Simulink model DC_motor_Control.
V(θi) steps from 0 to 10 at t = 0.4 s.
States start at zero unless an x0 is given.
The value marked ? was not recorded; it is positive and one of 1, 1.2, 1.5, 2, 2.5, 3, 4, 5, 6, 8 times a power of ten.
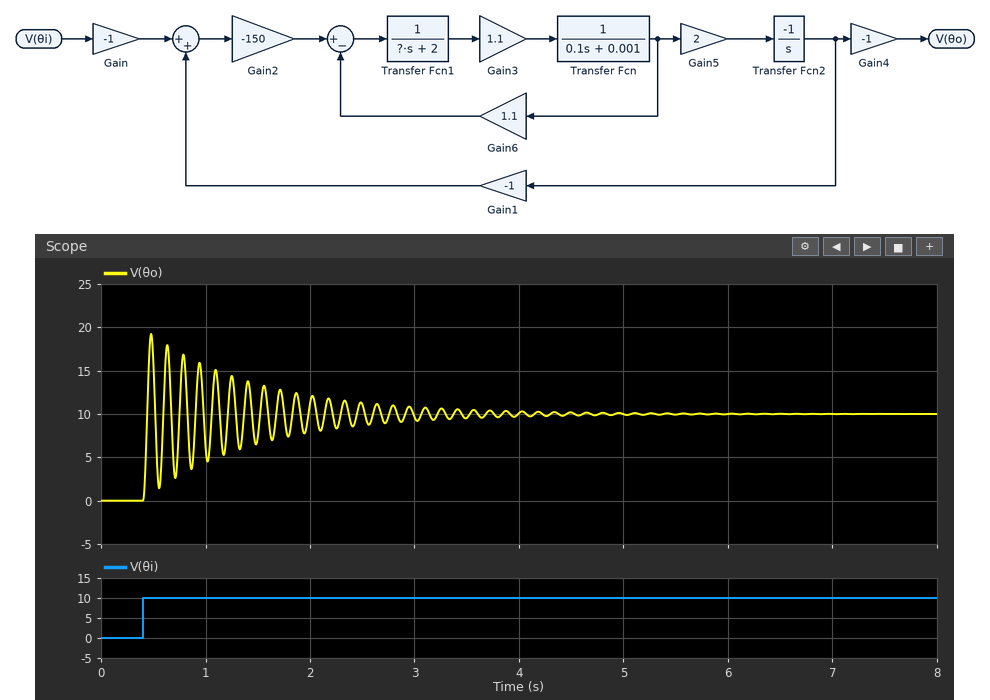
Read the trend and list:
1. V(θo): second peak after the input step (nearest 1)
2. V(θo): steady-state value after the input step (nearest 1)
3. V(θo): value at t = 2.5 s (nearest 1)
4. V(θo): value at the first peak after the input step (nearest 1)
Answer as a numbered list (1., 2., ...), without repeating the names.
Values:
1. 18
2. 10
3. 11
4. 19
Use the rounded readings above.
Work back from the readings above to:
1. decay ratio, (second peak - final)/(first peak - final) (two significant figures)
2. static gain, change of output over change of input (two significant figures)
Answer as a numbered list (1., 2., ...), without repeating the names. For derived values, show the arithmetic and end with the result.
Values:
1. (18 - 10) / (19 - 10) = 0.89
2. (10 - 0) / (10 - 0) = 1.0
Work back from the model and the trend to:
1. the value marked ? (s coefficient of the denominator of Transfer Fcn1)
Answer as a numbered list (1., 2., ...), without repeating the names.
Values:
1. 0.005
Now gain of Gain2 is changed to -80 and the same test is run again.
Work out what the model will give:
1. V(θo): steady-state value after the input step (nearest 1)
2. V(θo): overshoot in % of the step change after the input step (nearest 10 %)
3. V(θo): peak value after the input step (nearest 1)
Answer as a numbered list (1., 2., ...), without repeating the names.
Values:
1. 10
2. 80 %
3. 18
